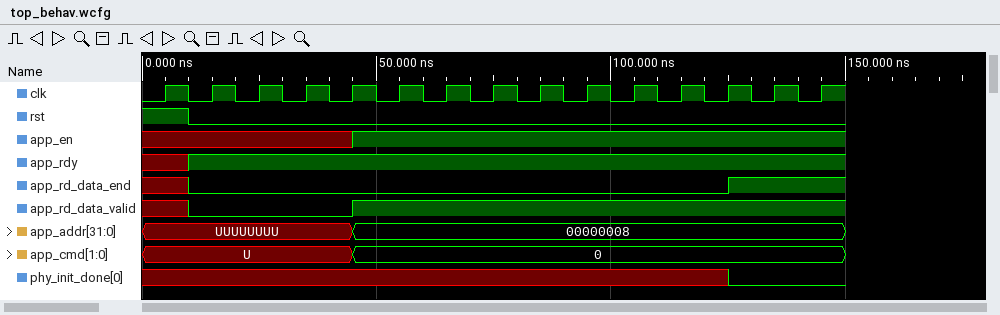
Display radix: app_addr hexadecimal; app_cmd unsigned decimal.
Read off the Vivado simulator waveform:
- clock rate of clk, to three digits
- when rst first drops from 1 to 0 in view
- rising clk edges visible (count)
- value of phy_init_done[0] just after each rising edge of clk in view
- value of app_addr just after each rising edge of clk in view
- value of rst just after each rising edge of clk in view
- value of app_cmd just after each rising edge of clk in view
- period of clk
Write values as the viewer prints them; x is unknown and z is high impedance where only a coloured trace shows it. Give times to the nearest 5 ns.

100 MHz
10 ns
15
x x x x x x x x x x x x 0 0 0
UUUUUUUU, UUUUUUUU, UUUUUUUU, UUUUUUUU, 00000008, 00000008, 00000008, 00000008, 00000008, 00000008, 00000008, 00000008, 00000008, 00000008, 00000008
1 0 0 0 0 0 0 0 0 0 0 0 0 0 0
U, U, U, U, 0, 0, 0, 0, 0, 0, 0, 0, 0, 0, 0
10 ns
